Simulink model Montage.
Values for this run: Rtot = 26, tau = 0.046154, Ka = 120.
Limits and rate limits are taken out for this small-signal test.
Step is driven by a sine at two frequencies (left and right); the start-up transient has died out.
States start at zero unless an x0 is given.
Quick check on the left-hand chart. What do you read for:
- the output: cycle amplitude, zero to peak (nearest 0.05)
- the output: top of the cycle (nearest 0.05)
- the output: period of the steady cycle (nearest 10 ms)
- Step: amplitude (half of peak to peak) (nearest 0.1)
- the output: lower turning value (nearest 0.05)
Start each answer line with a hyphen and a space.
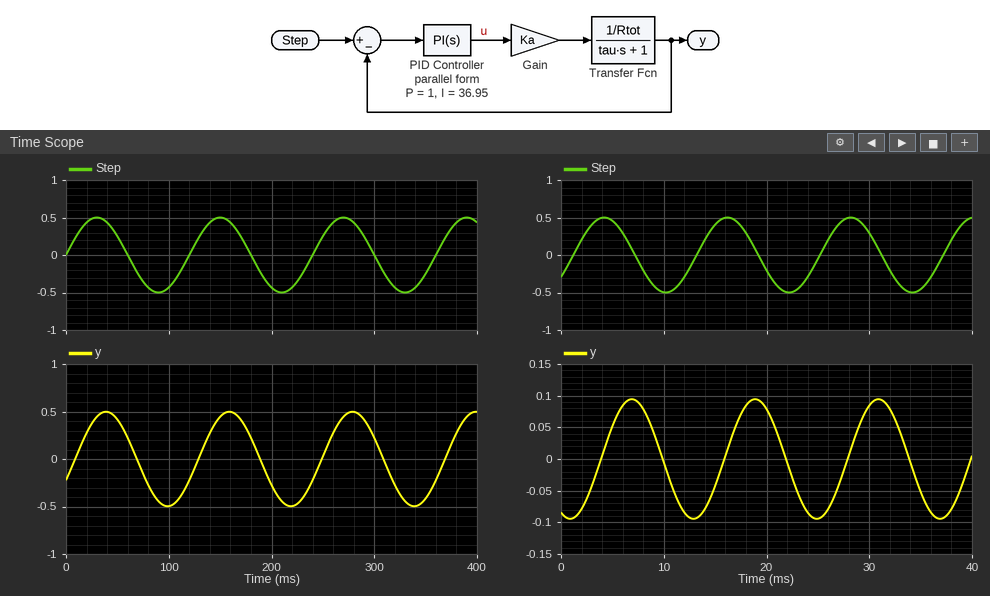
- 0.50
- 0.50
- 120 ms
- 0.5
- -0.50
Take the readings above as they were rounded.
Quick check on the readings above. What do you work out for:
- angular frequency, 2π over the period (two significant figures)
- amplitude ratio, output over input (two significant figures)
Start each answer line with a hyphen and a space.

- 0.052 rad/ms
- 1.0
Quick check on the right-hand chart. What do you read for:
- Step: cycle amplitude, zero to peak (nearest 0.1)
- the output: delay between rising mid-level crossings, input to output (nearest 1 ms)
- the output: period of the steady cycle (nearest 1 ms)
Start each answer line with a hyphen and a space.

- 0.5
- 3 ms
- 12 ms
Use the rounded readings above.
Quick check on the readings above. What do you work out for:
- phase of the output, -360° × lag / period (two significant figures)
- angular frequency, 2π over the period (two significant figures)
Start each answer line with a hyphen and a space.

- -90°
- 0.52 rad/ms
